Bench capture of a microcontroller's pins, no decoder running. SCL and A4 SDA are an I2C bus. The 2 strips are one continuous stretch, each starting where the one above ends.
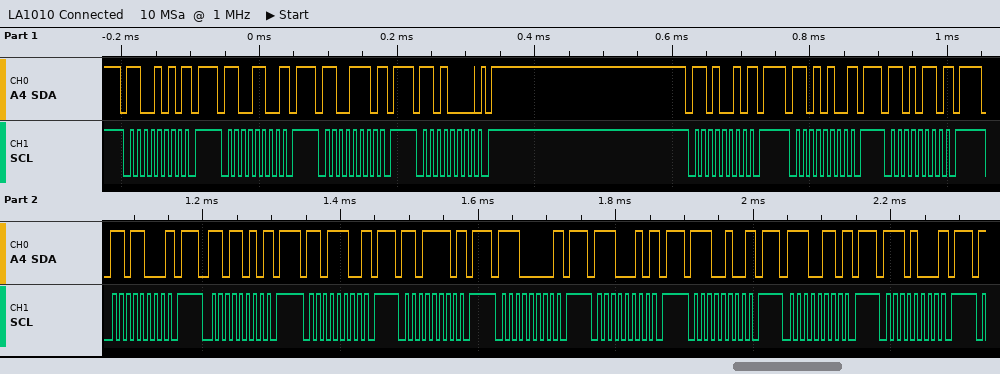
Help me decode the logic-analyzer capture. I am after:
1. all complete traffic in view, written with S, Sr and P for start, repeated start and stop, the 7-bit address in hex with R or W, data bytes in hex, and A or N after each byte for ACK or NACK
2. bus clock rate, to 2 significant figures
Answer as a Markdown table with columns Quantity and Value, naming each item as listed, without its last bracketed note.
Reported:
| Quantity | Value |
|---|---|
| all complete traffic in view, written with S, Sr and P for start, repeated start and stop, the 7-bit address in hex with R or W, data bytes in hex, and A or N after each byte for ACK or NACK | S 65W N P S 66W N P S 67W N P S 68W A P S 69W N P S 6AW N P S 6BW N P S 6CW N P S 6DW N P S 6EW N P S 6FW N P S 70W N P S 71W N P S 72W N P S 73W N P S 74W N P |
| bus clock rate, to 2 significant figures | 100 kHz |
